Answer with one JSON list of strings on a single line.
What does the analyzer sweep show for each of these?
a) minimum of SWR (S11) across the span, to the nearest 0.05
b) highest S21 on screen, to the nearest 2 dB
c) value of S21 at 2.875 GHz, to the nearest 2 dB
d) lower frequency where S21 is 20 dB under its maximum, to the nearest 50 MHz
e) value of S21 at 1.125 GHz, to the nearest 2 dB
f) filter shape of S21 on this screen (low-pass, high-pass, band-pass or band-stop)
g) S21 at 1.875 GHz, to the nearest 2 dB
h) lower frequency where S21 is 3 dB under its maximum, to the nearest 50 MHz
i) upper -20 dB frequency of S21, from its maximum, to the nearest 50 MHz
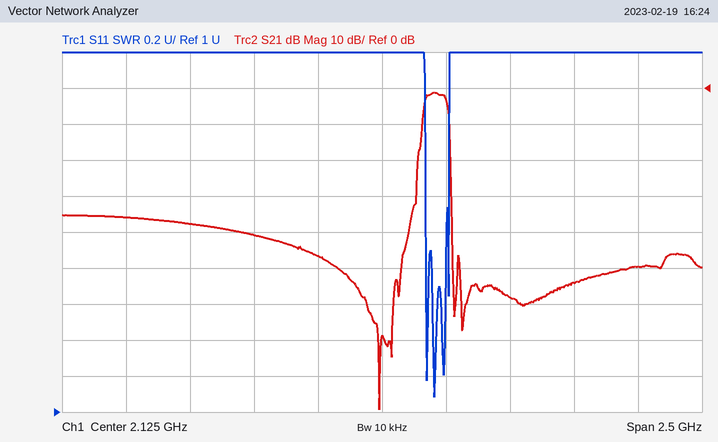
["1.10", "-2 dB", "-54 dB", "2.25 GHz", "-36 dB", "band-pass", "-46 dB", "2.30 GHz", "2.40 GHz"]
